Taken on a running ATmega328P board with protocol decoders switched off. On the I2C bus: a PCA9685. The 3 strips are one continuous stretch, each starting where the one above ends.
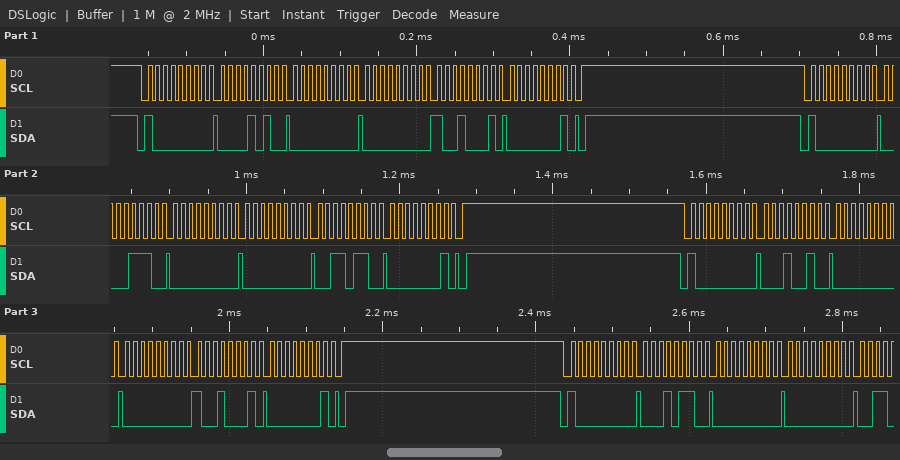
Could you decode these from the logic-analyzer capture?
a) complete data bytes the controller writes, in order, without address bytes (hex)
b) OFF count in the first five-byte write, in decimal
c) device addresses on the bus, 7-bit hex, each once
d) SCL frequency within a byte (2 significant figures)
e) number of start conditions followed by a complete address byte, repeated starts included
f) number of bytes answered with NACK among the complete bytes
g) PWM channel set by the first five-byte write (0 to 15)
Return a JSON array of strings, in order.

["0A 00 00 91 01 0E 00 00 36 01 12 00 00 91 01 16 00 00", "401", "0x40", "100 kHz", "4", "0", "1"]
